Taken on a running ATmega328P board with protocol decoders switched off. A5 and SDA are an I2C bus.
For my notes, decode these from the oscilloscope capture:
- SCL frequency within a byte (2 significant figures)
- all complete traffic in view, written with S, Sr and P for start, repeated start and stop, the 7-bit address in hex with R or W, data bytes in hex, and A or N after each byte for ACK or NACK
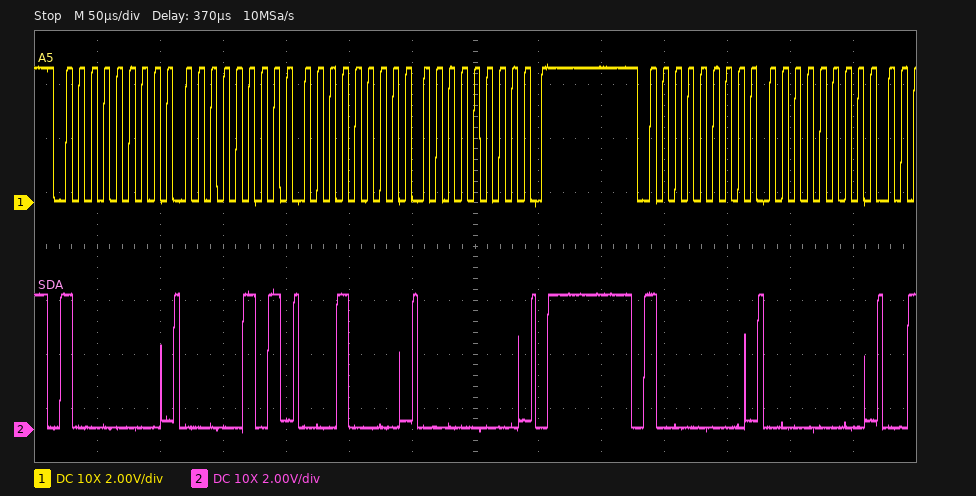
100 kHz
S 40W A 05 A 10 A 00 A P S 40W A 00 A
